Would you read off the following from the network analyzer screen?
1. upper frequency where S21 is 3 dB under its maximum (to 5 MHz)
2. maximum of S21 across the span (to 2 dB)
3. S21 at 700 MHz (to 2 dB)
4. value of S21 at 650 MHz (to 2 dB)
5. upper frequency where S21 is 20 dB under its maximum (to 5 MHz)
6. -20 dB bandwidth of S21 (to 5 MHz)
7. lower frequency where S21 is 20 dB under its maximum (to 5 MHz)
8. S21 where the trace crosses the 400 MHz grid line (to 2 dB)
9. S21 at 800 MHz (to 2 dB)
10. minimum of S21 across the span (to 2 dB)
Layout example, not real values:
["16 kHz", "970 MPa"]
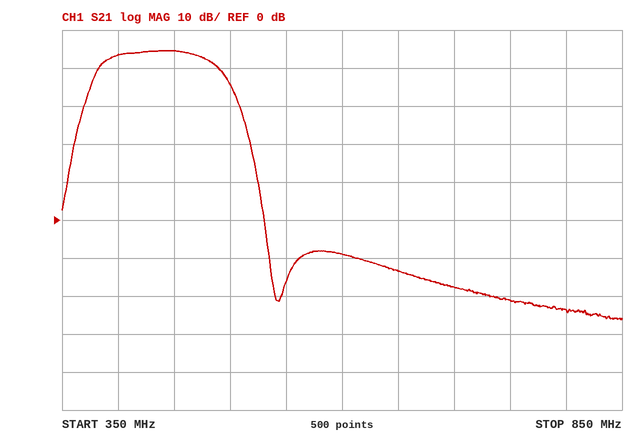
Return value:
["485 MHz", "44 dB", "-18 dB", "-14 dB", "515 MHz", "150 MHz", "365 MHz", "44 dB", "-24 dB", "-26 dB"]
